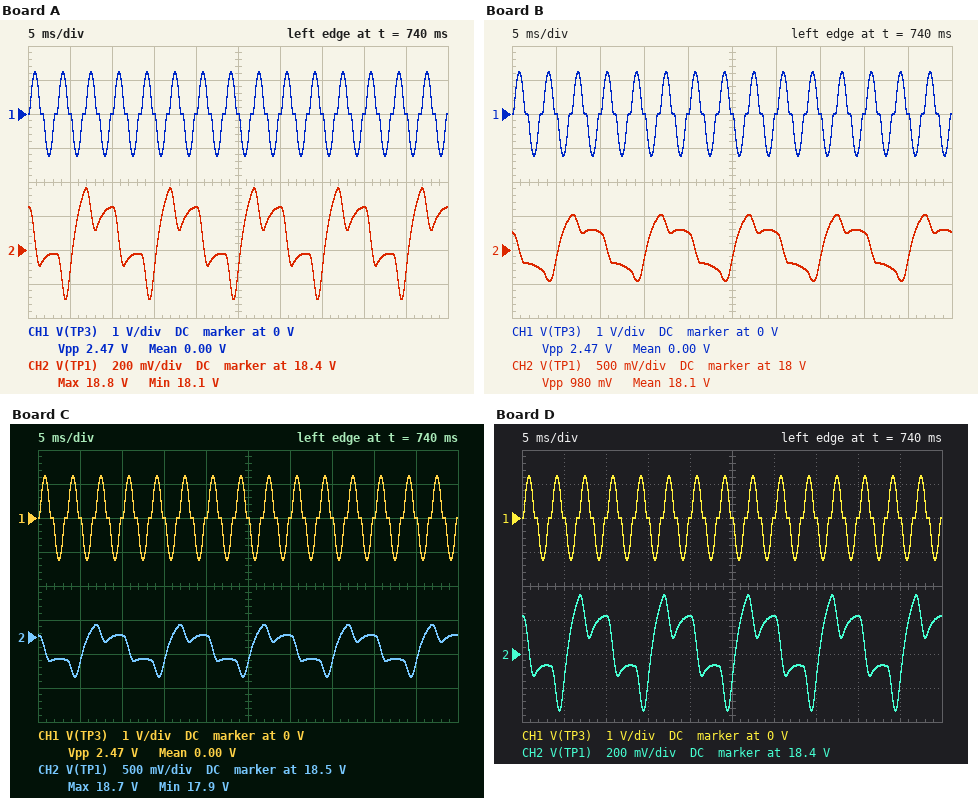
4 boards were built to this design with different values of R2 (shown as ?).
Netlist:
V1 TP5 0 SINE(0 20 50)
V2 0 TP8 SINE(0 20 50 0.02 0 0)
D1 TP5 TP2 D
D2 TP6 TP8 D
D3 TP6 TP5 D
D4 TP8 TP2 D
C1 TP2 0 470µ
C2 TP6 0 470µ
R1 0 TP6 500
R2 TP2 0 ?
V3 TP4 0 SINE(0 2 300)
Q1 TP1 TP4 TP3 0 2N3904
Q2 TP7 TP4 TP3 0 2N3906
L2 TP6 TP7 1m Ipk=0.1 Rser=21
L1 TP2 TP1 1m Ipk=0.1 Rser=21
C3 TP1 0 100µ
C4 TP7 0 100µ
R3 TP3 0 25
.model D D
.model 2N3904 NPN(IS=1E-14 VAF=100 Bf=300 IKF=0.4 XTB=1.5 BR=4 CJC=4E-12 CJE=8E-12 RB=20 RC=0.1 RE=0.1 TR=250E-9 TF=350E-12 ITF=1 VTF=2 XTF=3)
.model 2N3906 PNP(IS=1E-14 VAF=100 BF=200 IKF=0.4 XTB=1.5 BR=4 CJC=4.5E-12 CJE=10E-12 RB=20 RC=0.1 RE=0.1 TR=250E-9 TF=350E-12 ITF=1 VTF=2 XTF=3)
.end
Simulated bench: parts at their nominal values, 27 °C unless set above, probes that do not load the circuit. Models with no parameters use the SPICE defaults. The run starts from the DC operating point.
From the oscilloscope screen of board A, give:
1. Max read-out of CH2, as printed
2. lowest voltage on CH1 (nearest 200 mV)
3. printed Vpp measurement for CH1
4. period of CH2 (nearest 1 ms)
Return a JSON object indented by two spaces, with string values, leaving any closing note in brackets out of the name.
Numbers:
{
  "Max read-out of CH2, as printed": "18.8 V",
  "lowest voltage on CH1": "-1.2 V",
  "printed Vpp measurement for CH1": "2.47 V",
  "period of CH2": "10 ms"
}
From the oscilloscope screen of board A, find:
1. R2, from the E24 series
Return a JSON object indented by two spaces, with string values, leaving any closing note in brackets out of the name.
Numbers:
{
  "R2, from the E24 series": "470 Ω"
}
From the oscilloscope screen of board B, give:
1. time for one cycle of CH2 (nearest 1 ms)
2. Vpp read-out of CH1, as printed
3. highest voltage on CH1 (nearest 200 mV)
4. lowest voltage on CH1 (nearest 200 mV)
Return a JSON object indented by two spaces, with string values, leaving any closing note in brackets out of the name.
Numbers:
{
  "time for one cycle of CH2": "10 ms",
  "Vpp read-out of CH1, as printed": "2.47 V",
  "highest voltage on CH1": "1.2 V",
  "lowest voltage on CH1": "-1.2 V"
}
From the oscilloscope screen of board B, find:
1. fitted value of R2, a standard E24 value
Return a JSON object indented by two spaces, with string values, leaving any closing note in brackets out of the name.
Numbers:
{
  "fitted value of R2, a standard E24 value": "200 Ω"
}
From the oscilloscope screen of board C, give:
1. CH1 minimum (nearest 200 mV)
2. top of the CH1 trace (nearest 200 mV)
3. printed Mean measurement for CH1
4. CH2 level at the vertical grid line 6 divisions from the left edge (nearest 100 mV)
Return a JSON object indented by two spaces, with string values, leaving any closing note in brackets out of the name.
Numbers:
{
  "CH1 minimum": "-1.2 V",
  "top of the CH1 trace": "1.2 V",
  "printed Mean measurement for CH1": "0.00 V",
  "CH2 level at the vertical grid line 6 divisions from the left edge": "18.5 V"
}
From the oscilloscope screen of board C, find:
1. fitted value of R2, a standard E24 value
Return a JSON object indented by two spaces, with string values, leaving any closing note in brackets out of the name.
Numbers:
{
  "fitted value of R2, a standard E24 value": "330 Ω"
}
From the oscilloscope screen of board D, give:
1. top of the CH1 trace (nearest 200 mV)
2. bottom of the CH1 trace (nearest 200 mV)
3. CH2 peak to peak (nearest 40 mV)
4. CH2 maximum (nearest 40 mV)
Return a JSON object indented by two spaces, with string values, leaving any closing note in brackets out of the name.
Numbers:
{
  "top of the CH1 trace": "1.2 V",
  "bottom of the CH1 trace": "-1.2 V",
  "CH2 peak to peak": "680 mV",
  "CH2 maximum": "18.76 V"
}
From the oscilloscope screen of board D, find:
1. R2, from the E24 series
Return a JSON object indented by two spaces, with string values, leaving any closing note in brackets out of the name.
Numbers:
{
  "R2, from the E24 series": "430 Ω"
}
